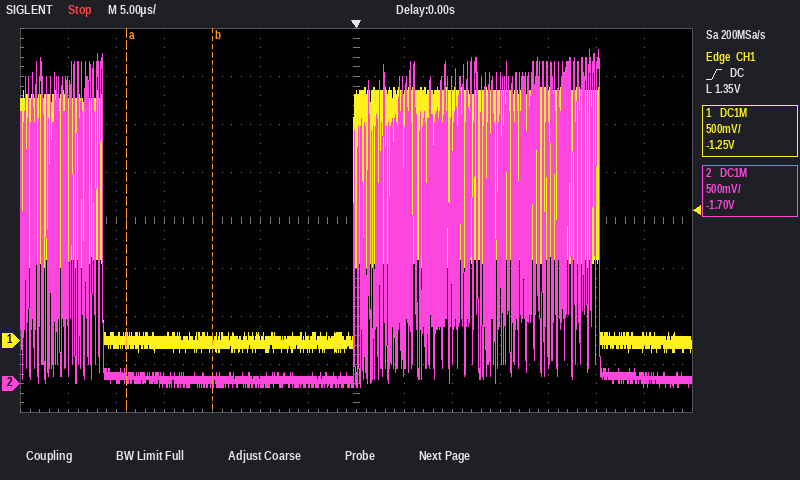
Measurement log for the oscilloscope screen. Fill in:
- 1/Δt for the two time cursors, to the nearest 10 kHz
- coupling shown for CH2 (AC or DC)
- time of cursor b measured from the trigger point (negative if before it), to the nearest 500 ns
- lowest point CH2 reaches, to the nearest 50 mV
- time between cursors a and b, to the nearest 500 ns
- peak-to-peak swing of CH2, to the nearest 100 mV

110 kHz
DC
-15.0 µs
-50 mV
9.0 µs
3.50 V
